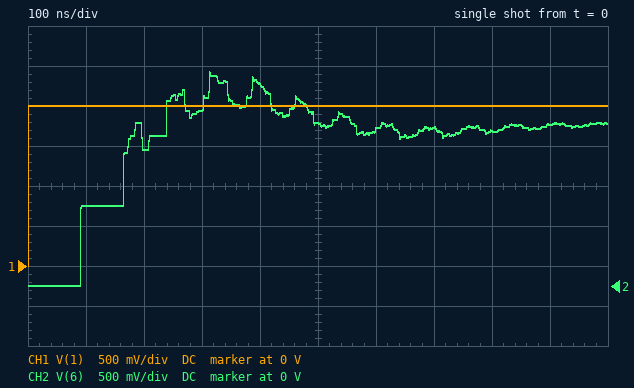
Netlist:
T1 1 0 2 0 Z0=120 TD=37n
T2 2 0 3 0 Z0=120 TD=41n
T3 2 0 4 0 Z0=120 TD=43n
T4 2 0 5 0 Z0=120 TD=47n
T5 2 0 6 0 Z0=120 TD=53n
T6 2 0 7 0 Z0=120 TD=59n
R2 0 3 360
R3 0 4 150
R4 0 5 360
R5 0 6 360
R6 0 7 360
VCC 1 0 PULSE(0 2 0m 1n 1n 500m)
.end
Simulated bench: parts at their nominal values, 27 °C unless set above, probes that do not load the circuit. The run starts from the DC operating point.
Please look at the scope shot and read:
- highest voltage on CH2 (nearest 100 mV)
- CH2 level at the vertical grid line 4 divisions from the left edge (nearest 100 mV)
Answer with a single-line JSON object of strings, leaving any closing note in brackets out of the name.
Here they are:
{"highest voltage on CH2": "2.7 V", "CH2 level at the vertical grid line 4 divisions from the left edge": "2.5 V"}
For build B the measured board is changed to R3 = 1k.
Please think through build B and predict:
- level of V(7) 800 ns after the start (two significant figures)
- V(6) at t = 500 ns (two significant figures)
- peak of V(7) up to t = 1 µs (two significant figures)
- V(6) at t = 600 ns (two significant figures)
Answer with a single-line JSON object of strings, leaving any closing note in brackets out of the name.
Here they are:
{"level of V(7) 800 ns after the start": "1.9 V", "V(6) at t = 500 ns": "2.1 V", "peak of V(7) up to t = 1 µs": "2.9 V", "V(6) at t = 600 ns": "1.8 V"}
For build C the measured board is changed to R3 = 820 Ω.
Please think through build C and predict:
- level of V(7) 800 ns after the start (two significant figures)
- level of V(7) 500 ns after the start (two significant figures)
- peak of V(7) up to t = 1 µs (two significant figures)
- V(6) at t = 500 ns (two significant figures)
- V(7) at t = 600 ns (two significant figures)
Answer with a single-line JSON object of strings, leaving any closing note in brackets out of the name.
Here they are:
{"level of V(7) 800 ns after the start": "1.9 V", "level of V(7) 500 ns after the start": "2.2 V", "peak of V(7) up to t = 1 µs": "2.9 V", "V(6) at t = 500 ns": "2.1 V", "V(7) at t = 600 ns": "1.7 V"}
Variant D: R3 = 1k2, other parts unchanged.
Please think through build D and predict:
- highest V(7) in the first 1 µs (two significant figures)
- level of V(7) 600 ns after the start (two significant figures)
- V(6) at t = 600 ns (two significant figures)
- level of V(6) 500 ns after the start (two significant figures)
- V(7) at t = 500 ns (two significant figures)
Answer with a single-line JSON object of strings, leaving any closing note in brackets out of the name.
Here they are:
{"highest V(7) in the first 1 µs": "2.9 V", "level of V(7) 600 ns after the start": "1.7 V", "V(6) at t = 600 ns": "1.8 V", "level of V(6) 500 ns after the start": "2.1 V", "V(7) at t = 500 ns": "2.2 V"}
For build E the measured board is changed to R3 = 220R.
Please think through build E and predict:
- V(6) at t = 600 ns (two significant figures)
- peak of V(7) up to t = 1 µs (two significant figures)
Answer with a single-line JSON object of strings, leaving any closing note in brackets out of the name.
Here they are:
{"V(6) at t = 600 ns": "1.9 V", "peak of V(7) up to t = 1 µs": "2.7 V"}
